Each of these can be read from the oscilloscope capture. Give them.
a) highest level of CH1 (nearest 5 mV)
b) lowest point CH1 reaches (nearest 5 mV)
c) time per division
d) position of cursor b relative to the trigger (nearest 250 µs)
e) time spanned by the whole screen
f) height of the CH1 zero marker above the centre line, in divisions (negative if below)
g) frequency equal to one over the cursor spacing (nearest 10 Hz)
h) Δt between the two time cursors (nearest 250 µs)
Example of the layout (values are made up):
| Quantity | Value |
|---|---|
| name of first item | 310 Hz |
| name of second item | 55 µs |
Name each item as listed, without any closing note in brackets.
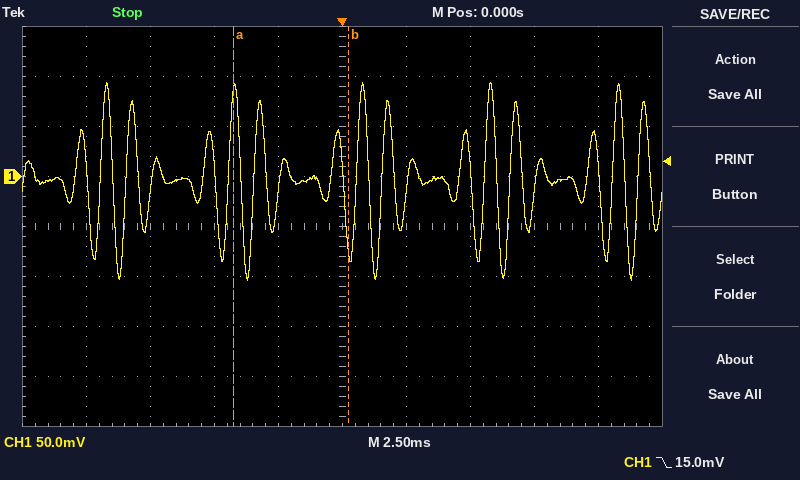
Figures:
| Quantity | Value |
|---|---|
| highest level of CH1 | 95 mV |
| lowest point CH1 reaches | -105 mV |
| time per division | 2.5 ms |
| position of cursor b relative to the trigger | +250 µs |
| time spanned by the whole screen | 25 ms |
| height of the CH1 zero marker above the centre line, in divisions | +1.0 div |
| frequency equal to one over the cursor spacing | 220 Hz |
| Δt between the two time cursors | 4.50 ms |
